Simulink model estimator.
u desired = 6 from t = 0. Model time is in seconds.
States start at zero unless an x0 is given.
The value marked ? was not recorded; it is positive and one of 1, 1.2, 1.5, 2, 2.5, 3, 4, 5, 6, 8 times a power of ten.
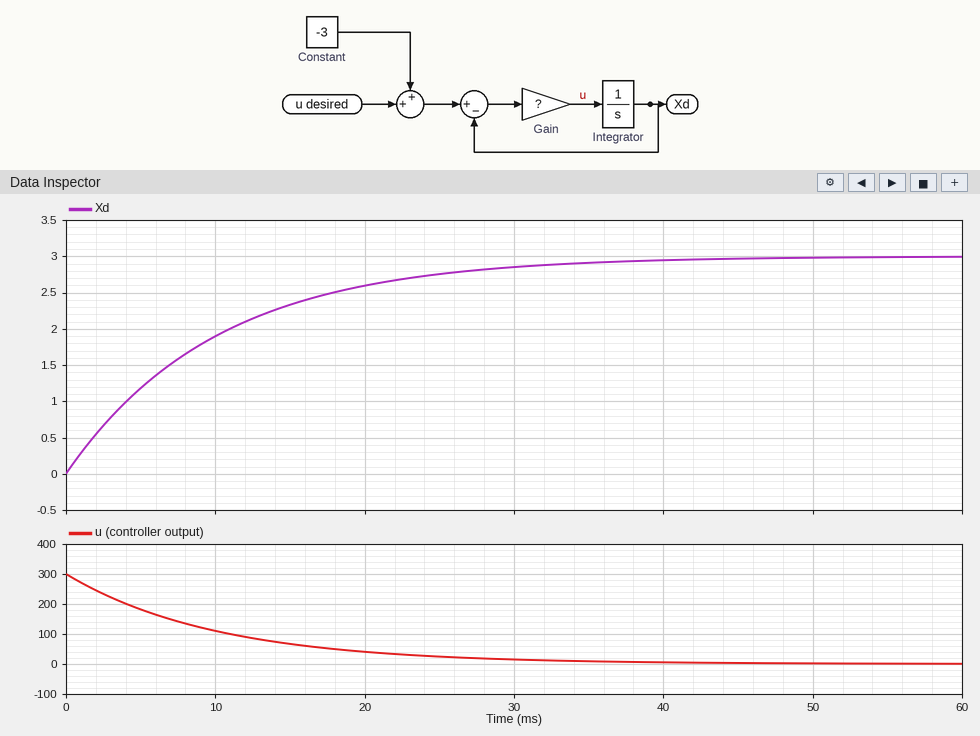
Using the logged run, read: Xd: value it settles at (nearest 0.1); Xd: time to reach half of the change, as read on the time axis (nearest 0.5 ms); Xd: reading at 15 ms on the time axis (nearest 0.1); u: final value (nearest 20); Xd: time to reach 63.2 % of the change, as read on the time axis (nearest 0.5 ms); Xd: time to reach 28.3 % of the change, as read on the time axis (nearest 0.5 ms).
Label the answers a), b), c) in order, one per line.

a) 3.0
b) 7.0 ms
c) 2.3
d) 0
e) 10.0 ms
f) 3.5 ms
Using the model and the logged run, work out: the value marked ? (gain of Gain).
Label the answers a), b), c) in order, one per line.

a) 100
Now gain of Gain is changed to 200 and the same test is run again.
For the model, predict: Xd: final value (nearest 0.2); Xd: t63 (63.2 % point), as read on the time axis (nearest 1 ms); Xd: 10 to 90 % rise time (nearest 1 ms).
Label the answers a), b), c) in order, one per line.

a) 3.0
b) 5 ms
c) 11 ms
